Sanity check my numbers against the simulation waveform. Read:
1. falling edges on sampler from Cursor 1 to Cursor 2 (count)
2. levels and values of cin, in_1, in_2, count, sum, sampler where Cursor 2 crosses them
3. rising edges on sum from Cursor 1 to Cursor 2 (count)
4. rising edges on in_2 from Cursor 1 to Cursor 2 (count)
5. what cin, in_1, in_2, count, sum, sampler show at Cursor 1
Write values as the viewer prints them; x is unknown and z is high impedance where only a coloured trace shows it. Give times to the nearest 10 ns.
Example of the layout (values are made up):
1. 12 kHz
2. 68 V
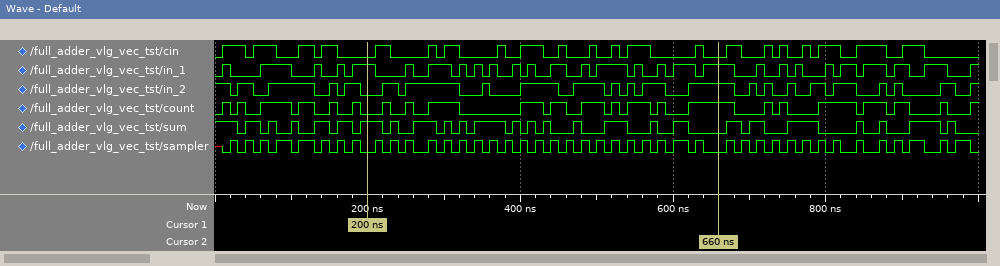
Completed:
1. 21
2. cin=0, in_1=1, in_2=1, count=1, sum=0, sampler=0
3. 12
4. 9
5. cin=0, in_1=1, in_2=0, count=0, sum=1, sampler=0
